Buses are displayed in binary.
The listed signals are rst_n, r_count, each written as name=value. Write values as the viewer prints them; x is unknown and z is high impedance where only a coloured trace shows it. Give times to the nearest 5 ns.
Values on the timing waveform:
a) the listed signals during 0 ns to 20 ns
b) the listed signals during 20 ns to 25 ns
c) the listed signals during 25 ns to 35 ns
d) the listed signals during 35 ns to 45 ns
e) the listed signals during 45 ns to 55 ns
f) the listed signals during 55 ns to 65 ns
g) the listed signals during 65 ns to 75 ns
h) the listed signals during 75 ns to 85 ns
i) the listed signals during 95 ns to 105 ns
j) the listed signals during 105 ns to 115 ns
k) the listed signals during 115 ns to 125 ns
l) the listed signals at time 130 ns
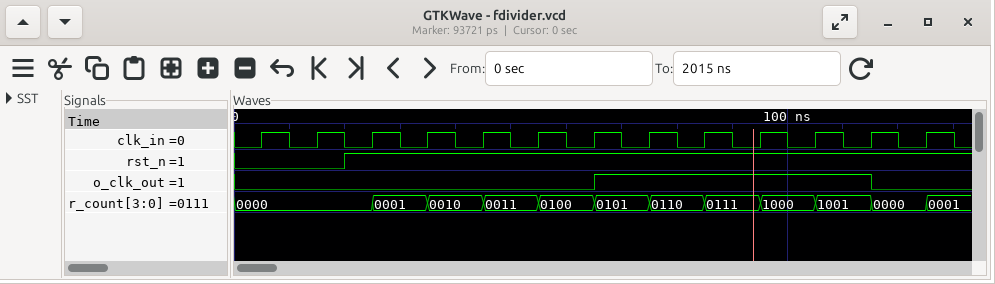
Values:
rst_n=0, r_count=0000
rst_n=1, r_count=0000
rst_n=1, r_count=0001
rst_n=1, r_count=0010
rst_n=1, r_count=0011
rst_n=1, r_count=0100
rst_n=1, r_count=0101
rst_n=1, r_count=0110
rst_n=1, r_count=1000
rst_n=1, r_count=1001
rst_n=1, r_count=0000
rst_n=1, r_count=0001
